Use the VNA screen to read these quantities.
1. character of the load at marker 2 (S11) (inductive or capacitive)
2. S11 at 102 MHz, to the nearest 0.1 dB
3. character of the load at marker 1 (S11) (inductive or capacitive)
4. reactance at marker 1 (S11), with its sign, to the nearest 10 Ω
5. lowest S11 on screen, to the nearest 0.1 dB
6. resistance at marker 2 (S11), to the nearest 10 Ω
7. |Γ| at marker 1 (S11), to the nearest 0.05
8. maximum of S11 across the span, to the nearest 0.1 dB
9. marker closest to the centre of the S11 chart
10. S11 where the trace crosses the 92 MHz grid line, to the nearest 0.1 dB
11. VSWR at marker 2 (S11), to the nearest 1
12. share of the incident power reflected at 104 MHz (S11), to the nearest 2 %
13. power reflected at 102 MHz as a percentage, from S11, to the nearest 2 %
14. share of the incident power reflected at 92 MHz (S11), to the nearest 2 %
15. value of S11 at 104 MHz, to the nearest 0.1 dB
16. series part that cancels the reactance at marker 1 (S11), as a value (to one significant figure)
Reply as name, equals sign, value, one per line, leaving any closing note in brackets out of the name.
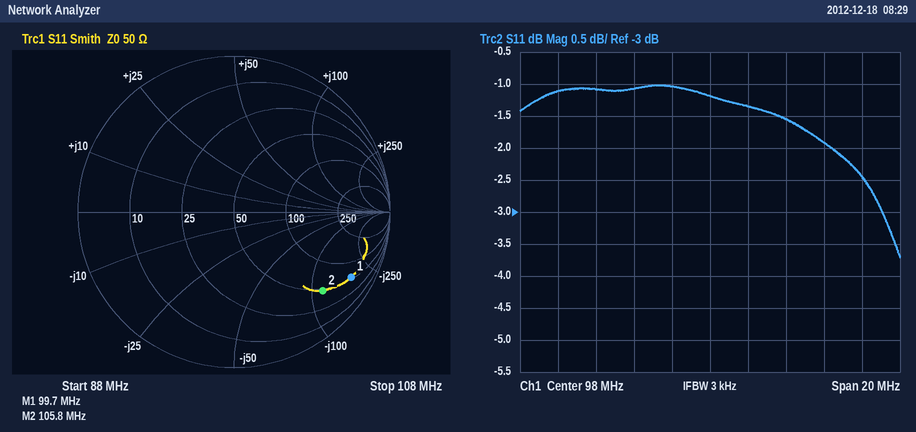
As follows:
character of the load at marker 2 (S11) = capacitive
S11 at 102 MHz, to the nearest 0.1 dB = -1.5 dB
character of the load at marker 1 (S11) = capacitive
reactance at marker 1 (S11), with its sign, to the nearest 10 Ω = -180 Ω
lowest S11 on screen, to the nearest 0.1 dB = -3.7 dB
resistance at marker 2 (S11), to the nearest 10 Ω = 50 Ω
|Γ| at marker 1 (S11), to the nearest 0.05 = 0.85
maximum of S11 across the span, to the nearest 0.1 dB = -1.0 dB
marker closest to the centre of the S11 chart = marker 2
S11 where the trace crosses the 92 MHz grid line, to the nearest 0.1 dB = -1.1 dB
VSWR at marker 2 (S11), to the nearest 1 = 7
share of the incident power reflected at 104 MHz (S11), to the nearest 2 % = 64 %
power reflected at 102 MHz as a percentage, from S11, to the nearest 2 % = 70 %
share of the incident power reflected at 92 MHz (S11), to the nearest 2 % = 78 %
value of S11 at 104 MHz, to the nearest 0.1 dB = -1.9 dB
series part that cancels the reactance at marker 1 (S11), as a value = 300 nH
